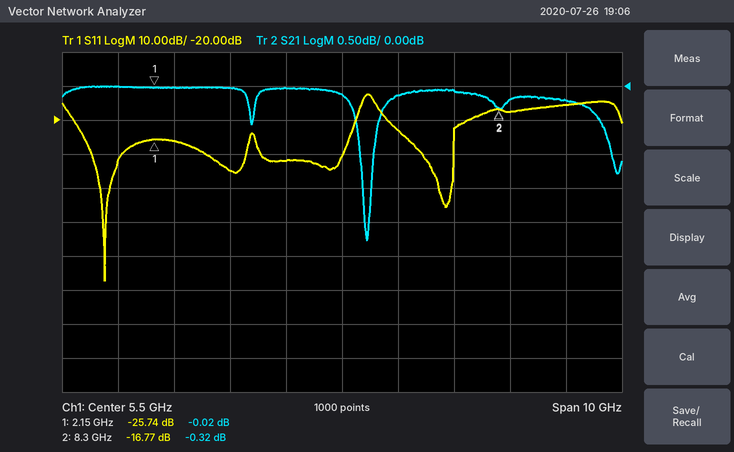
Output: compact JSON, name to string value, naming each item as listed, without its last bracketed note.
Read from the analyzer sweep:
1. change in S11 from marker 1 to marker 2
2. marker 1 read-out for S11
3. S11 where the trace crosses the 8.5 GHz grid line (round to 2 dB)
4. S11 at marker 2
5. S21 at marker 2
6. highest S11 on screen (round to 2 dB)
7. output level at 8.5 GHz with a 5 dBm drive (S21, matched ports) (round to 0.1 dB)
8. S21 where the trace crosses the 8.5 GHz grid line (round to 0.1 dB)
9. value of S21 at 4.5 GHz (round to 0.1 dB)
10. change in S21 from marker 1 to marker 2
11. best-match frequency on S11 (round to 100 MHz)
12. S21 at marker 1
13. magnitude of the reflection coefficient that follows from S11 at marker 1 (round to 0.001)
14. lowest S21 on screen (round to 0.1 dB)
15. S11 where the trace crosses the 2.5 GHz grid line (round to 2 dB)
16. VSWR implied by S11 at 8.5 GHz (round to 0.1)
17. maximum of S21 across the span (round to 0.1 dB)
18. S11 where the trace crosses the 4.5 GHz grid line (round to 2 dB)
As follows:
{"change in S11 from marker 1 to marker 2": "8.97 dB", "marker 1 read-out for S11": "-25.74 dB", "S11 where the trace crosses the 8.5 GHz grid line": "-18 dB", "S11 at marker 2": "-16.77 dB", "S21 at marker 2": "-0.32 dB", "highest S11 on screen": "-12 dB", "output level at 8.5 GHz with a 5 dBm drive (S21, matched ports)": "4.8 dBm", "S21 where the trace crosses the 8.5 GHz grid line": "-0.2 dB", "value of S21 at 4.5 GHz": "0.0 dB", "change in S21 from marker 1 to marker 2": "-0.30 dB", "best-match frequency on S11": "1.3 GHz", "S21 at marker 1": "-0.02 dB", "magnitude of the reflection coefficient that follows from S11 at marker 1": "0.052", "lowest S21 on screen": "-2.3 dB", "S11 where the trace crosses the 2.5 GHz grid line": "-26 dB", "VSWR implied by S11 at 8.5 GHz": "1.3", "maximum of S21 across the span": "0.0 dB", "S11 where the trace crosses the 4.5 GHz grid line": "-32 dB"}
